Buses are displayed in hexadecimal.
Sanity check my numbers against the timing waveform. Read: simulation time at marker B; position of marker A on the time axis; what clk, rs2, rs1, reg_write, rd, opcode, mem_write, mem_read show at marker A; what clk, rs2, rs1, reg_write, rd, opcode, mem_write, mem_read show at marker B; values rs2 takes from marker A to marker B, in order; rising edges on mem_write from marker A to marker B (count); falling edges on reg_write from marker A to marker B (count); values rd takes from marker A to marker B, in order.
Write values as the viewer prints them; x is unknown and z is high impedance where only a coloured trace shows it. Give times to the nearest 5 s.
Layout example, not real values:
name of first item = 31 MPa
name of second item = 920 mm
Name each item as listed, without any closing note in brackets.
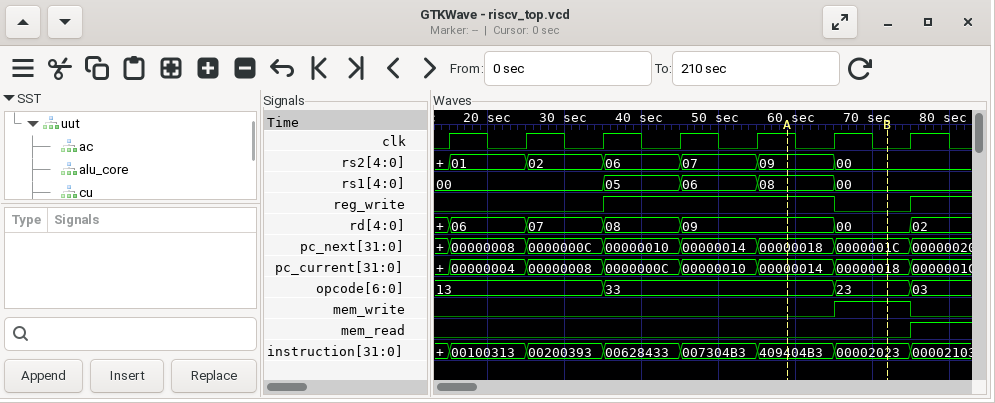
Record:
simulation time at marker B = 70 s
position of marker A on the time axis = 60 s
what clk, rs2, rs1, reg_write, rd, opcode, mem_write, mem_read show at marker A = clk=1, rs2=09, rs1=08, reg_write=1, rd=09, opcode=33, mem_write=0, mem_read=0
what clk, rs2, rs1, reg_write, rd, opcode, mem_write, mem_read show at marker B = clk=0, rs2=00, rs1=00, reg_write=0, rd=00, opcode=23, mem_write=1, mem_read=0
values rs2 takes from marker A to marker B, in order = 09, 00
rising edges on mem_write from marker A to marker B = 1
falling edges on reg_write from marker A to marker B = 1
values rd takes from marker A to marker B, in order = 09, 00
